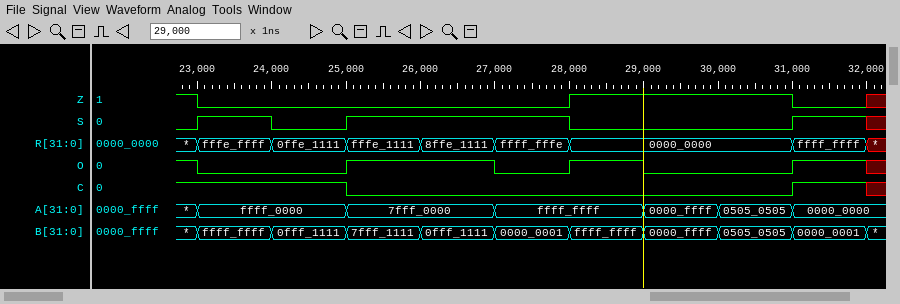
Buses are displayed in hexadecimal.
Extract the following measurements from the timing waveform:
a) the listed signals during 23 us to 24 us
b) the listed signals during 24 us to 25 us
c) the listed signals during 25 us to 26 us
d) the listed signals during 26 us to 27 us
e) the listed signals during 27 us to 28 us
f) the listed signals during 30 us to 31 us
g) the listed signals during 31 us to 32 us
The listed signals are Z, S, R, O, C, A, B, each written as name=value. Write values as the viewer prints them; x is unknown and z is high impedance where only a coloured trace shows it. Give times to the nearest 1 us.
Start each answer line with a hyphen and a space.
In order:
- Z=0, S=1, R=fffe_ffff, O=0, C=1, A=ffff_0000, B=ffff_ffff
- Z=0, S=0, R=0ffe_1111, O=0, C=1, A=ffff_0000, B=0fff_1111
- Z=0, S=1, R=fffe_1111, O=1, C=0, A=7fff_0000, B=7fff_1111
- Z=0, S=1, R=8ffe_1111, O=1, C=0, A=7fff_0000, B=0fff_1111
- Z=0, S=1, R=ffff_fffe, O=0, C=0, A=ffff_ffff, B=0000_0001
- Z=1, S=0, R=0000_0000, O=0, C=0, A=0505_0505, B=0505_0505
- Z=0, S=1, R=ffff_ffff, O=1, C=1, A=0000_0000, B=0000_0001
